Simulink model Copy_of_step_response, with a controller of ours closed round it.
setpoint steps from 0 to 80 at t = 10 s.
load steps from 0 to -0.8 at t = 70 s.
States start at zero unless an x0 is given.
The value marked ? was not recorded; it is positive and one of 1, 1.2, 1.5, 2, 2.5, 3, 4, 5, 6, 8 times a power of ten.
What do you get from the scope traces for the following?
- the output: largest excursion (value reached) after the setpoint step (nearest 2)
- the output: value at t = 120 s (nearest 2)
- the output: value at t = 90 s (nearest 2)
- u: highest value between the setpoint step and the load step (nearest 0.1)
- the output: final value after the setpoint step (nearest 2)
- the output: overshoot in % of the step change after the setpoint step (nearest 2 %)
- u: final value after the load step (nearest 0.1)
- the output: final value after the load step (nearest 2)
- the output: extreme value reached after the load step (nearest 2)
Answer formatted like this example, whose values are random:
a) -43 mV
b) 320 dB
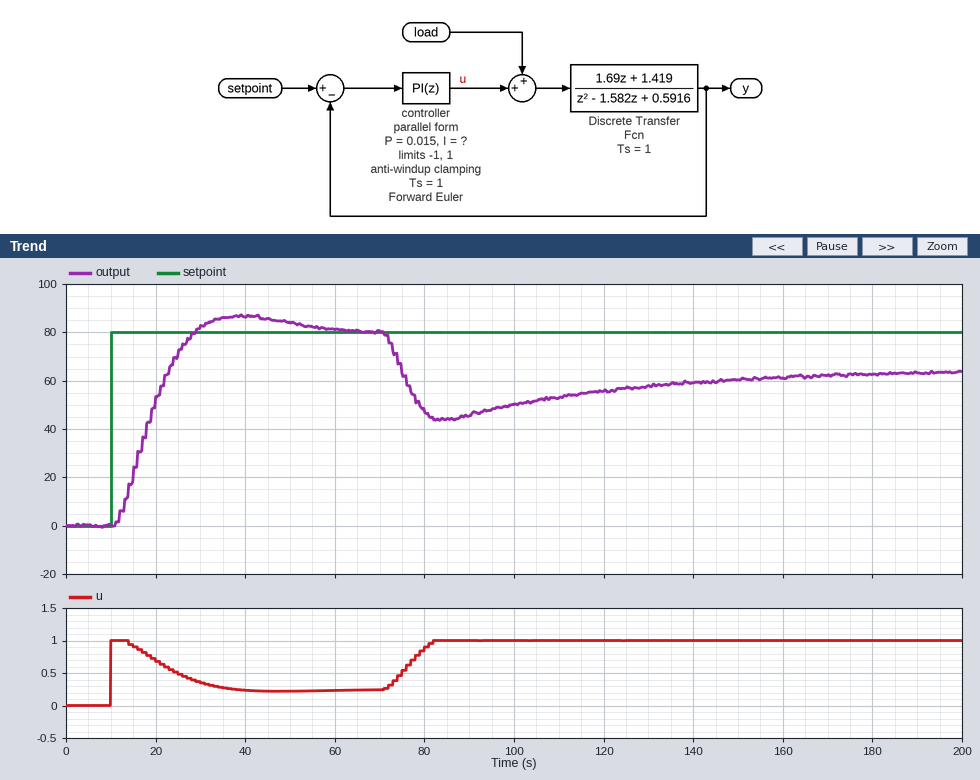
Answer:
a) 86
b) 56
c) 46
d) 1.0
e) 80
f) 8 %
g) 1.0
h) 64
i) 44
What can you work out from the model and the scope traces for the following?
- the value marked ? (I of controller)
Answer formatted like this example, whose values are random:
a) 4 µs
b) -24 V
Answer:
a) 0.001
